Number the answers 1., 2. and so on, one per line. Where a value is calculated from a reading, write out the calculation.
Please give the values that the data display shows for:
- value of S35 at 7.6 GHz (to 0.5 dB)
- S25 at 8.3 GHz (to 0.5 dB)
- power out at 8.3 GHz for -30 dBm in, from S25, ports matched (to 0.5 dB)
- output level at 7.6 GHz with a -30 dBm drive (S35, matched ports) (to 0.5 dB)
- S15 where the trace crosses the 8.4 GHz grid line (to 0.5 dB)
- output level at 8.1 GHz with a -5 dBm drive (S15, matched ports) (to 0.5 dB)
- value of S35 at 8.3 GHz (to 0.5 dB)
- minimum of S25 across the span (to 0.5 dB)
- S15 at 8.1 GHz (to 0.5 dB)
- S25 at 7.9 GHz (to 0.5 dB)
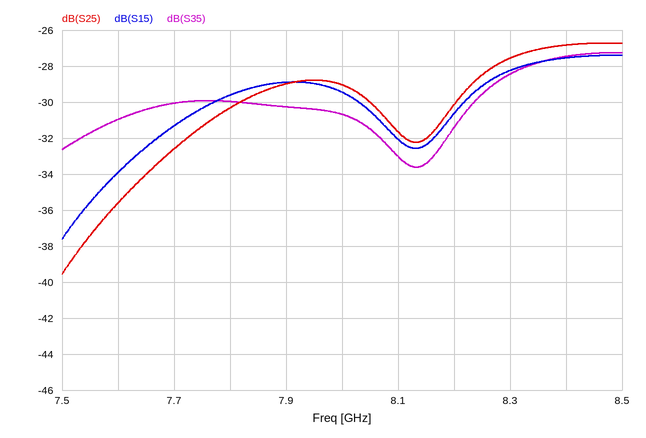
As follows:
1. -31.0 dB
2. -27.5 dB
3. -30 dBm + (-27.5 dB) = -57.5 dBm
4. -30 dBm + (-31.0 dB) = -61.0 dBm
5. -27.5 dB
6. -5 dBm + (-32.0 dB) = -37.0 dBm
7. -28.5 dB
8. -39.5 dB
9. -32.0 dB
10. -29.0 dB
